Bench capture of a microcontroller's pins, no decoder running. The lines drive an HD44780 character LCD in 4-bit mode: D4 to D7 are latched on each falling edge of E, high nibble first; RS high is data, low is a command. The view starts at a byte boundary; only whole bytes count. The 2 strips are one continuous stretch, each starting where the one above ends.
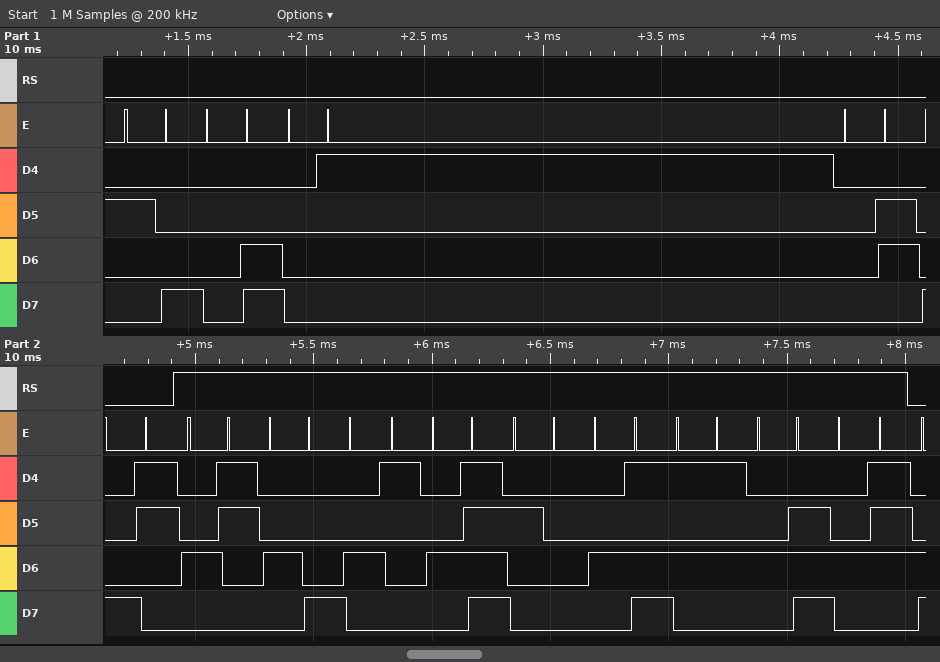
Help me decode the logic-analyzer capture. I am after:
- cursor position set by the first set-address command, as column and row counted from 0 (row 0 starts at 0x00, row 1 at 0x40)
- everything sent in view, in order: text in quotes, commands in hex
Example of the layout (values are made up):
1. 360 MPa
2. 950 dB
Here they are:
1. column 3, row 0
2. 0x28 0x0C 0x01 0x06 0x83 "CHAO MUNG"
